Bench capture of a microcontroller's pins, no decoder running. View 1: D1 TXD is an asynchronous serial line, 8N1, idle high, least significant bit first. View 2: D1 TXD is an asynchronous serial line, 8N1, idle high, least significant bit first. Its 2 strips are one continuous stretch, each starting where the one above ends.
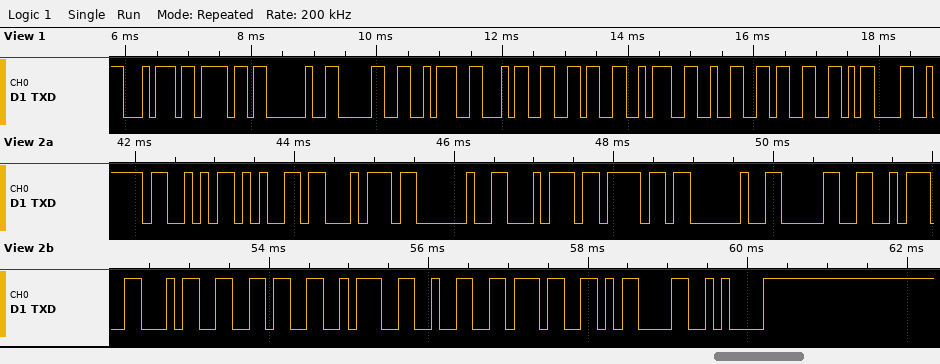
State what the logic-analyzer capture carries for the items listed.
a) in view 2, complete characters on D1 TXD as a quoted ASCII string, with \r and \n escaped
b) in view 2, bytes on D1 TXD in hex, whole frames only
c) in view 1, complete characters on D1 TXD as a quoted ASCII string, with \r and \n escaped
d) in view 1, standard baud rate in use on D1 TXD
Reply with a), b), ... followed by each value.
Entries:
a) "Set to 0:46:27\r\n"
b) 53 65 74 20 74 6F 20 30 3A 34 36 3A 32 37 0D 0A
c) "to 0:46:23\r"
d) 9600 baud
